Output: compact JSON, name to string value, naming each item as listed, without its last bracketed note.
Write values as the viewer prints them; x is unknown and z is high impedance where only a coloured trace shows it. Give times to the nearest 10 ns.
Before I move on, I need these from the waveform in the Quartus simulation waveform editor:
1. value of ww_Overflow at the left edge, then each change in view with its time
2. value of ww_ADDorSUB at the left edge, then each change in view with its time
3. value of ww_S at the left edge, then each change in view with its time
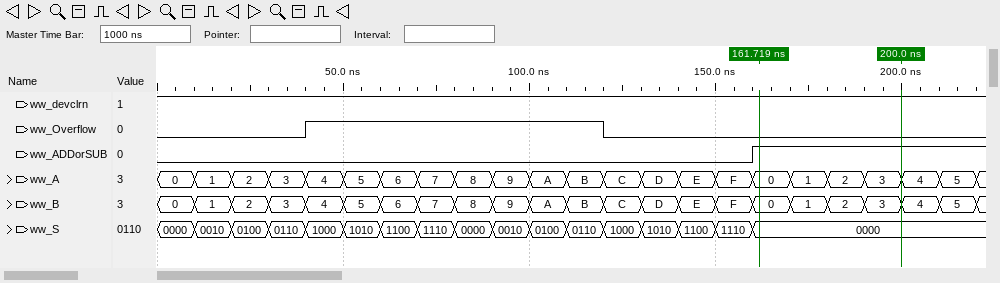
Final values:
{"value of ww_Overflow at the left edge, then each change in view with its time": "0, 1 at 40 ns, 0 at 120 ns", "value of ww_ADDorSUB at the left edge, then each change in view with its time": "0, 1 at 160 ns", "value of ww_S at the left edge, then each change in view with its time": "0000, 0010 at 10 ns, 0100 at 20 ns, 0110 at 30 ns, 1000 at 40 ns, 1010 at 50 ns, 1100 at 60 ns, 1110 at 70 ns, 0000 at 80 ns, 0010 at 90 ns, 0100 at 100 ns, 0110 at 110 ns, 1000 at 120 ns, 1010 at 130 ns, 1100 at 140 ns, 1110 at 150 ns, 0000 at 160 ns"}
